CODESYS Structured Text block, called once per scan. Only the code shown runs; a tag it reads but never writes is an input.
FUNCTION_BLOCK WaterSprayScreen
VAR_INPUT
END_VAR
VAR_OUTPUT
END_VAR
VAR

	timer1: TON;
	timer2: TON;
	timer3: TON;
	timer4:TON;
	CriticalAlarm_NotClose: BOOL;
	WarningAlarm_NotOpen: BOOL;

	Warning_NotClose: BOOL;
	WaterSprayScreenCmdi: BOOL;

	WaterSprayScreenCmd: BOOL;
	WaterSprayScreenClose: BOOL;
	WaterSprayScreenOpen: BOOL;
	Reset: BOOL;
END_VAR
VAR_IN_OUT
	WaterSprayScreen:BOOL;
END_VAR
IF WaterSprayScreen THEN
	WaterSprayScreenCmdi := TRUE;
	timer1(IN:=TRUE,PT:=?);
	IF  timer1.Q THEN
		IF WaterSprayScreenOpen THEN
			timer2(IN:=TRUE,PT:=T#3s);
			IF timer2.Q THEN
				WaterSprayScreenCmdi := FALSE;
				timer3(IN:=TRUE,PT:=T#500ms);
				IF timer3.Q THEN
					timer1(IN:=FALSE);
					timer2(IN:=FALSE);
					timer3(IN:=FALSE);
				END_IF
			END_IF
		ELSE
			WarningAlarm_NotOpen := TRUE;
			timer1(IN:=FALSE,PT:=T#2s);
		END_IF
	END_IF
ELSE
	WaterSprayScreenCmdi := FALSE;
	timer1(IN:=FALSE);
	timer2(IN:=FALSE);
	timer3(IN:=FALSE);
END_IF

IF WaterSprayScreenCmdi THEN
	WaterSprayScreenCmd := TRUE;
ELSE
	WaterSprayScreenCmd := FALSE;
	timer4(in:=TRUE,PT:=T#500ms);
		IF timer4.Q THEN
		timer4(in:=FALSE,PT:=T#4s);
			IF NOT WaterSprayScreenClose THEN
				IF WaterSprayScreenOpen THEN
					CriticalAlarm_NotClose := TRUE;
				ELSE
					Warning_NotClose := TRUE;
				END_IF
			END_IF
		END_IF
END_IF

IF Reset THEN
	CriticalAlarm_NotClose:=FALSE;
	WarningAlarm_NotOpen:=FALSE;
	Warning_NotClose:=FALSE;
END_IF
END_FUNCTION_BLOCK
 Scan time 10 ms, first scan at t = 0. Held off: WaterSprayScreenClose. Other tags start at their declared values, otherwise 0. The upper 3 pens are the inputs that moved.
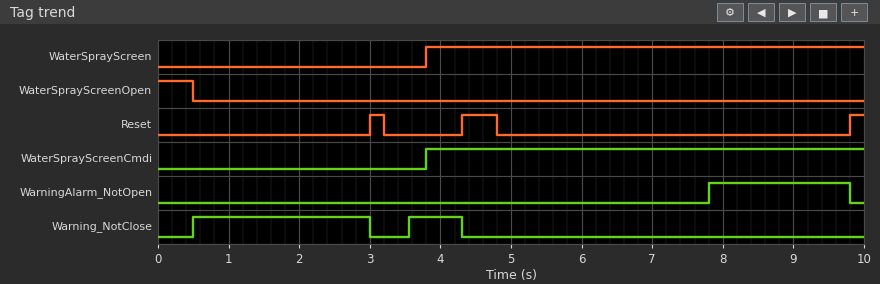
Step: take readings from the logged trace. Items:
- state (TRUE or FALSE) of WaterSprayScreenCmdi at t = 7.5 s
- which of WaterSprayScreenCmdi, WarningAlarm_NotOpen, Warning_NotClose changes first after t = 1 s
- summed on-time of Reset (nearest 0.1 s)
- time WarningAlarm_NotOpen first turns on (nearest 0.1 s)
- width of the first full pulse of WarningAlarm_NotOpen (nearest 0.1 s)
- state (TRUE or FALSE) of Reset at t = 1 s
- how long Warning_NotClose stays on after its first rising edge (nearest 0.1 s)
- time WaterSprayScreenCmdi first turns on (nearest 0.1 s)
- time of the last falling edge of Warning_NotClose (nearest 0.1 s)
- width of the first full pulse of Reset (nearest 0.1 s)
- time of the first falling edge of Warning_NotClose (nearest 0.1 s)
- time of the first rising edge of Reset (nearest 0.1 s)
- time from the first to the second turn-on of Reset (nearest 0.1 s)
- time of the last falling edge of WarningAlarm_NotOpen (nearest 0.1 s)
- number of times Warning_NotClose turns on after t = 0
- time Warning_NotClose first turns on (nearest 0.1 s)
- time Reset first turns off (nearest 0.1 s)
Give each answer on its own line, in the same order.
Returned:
TRUE
Warning_NotClose
0.9 s
7.8 s
2.0 s
FALSE
2.5 s
3.8 s
4.3 s
0.2 s
3.0 s
3.0 s
1.3 s
9.8 s
2
0.5 s
3.2 s
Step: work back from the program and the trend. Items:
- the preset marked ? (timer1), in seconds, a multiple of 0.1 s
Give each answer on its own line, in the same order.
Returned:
4.0 s
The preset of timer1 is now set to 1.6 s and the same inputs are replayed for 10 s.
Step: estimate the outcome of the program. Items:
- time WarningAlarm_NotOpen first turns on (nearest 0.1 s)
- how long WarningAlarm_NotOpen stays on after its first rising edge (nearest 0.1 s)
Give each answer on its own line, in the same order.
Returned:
5.4 s
4.4 s
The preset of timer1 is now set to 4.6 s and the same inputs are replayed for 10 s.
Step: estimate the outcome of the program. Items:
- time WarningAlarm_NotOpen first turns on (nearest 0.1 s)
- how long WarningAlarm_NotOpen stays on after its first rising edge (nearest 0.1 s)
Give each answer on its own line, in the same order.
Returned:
8.4 s
1.4 s
